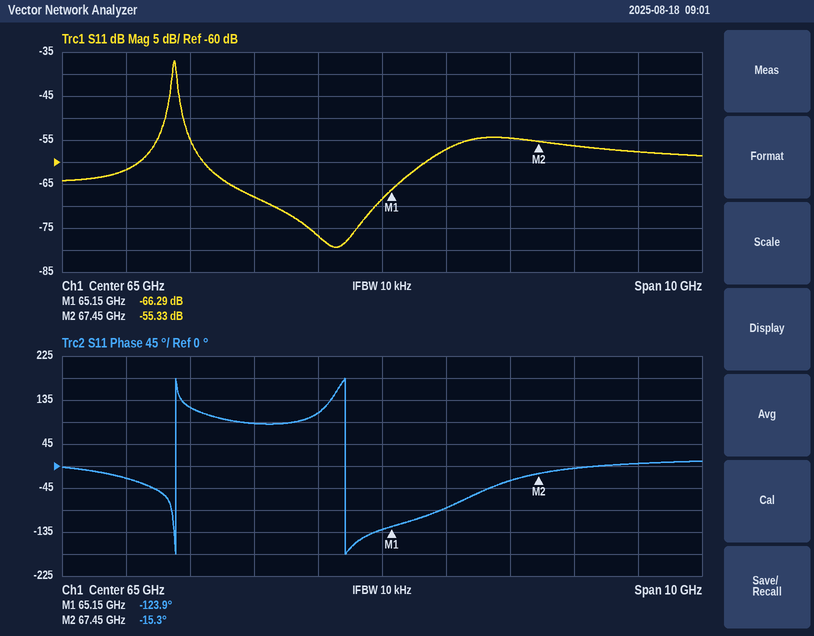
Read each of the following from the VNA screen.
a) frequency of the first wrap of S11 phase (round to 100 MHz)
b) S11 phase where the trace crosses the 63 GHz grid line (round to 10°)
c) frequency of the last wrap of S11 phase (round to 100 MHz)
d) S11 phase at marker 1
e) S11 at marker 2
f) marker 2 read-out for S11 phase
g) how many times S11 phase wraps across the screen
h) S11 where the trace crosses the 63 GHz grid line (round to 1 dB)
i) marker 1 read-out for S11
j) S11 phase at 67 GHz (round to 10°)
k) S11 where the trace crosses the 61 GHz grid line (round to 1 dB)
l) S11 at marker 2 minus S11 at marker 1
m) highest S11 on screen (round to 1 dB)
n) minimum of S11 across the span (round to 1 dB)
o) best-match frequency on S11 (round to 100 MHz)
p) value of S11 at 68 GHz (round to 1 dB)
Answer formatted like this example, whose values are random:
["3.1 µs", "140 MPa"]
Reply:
["61.8 GHz", "90°", "64.4 GHz", "-123.9°", "-55.33 dB", "-15.3°", "2", "-68 dB", "-66.29 dB", "-30°", "-62 dB", "10.96 dB", "-37 dB", "-79 dB", "64.3 GHz", "-56 dB"]
